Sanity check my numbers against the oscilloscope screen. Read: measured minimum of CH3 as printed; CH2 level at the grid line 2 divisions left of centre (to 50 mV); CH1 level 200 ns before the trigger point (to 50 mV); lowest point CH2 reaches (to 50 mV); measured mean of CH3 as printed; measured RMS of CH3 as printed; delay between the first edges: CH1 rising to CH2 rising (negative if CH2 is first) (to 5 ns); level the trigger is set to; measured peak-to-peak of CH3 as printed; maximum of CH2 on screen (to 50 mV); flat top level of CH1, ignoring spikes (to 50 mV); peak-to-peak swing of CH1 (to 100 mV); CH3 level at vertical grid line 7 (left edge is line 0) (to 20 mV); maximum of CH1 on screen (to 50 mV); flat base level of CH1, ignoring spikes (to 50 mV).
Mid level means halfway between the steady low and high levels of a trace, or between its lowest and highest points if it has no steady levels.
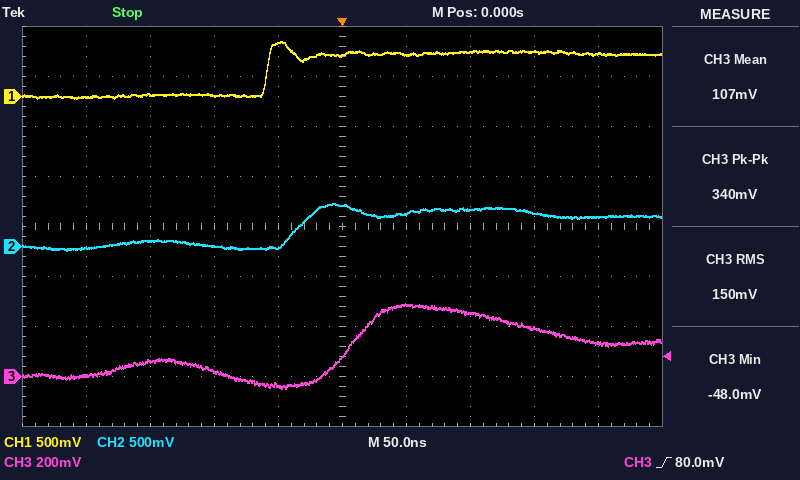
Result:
-48.0 mV
0 mV
0 mV
-50 mV
107 mV
150 mV
+25 ns
80.0 mV
340 mV
450 mV
450 mV
600 mV
260 mV
550 mV
0 mV
